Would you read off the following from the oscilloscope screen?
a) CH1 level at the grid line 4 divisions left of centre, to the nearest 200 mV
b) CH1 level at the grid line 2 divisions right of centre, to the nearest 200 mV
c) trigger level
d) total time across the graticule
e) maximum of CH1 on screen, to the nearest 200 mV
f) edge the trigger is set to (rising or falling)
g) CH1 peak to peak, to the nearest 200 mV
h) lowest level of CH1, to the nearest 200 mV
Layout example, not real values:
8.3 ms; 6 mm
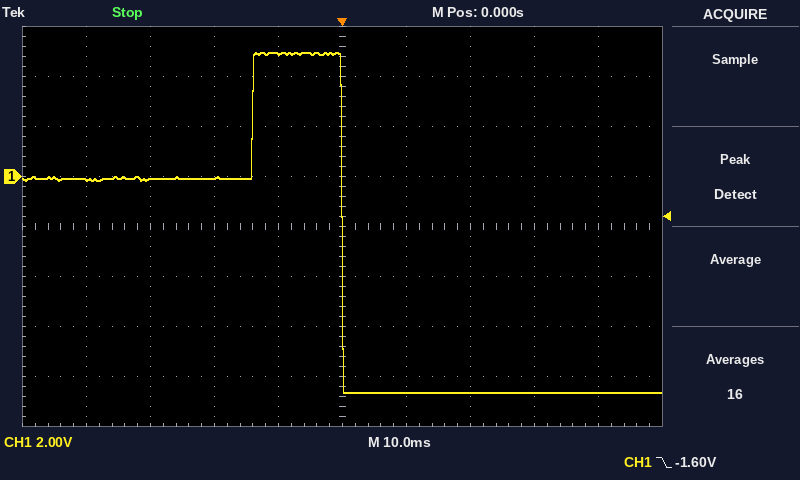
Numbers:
-200 mV; -8.6 V; -1.60 V; 100 ms; 5.0 V; falling; 13.6 V; -8.6 V
